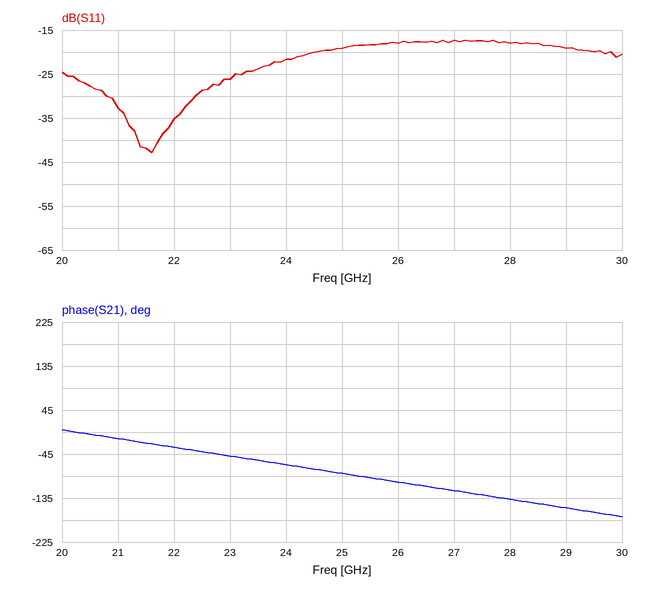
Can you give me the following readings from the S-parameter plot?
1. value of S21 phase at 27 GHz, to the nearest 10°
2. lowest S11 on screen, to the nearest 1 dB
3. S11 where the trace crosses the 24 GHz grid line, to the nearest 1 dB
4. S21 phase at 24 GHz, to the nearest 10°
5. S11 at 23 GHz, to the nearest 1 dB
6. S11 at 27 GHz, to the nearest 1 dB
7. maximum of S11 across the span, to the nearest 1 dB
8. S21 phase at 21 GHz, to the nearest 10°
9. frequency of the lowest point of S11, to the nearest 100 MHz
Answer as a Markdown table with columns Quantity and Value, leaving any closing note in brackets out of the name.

| Quantity | Value |
|---|---|
| value of S21 phase at 27 GHz, to the nearest 10° | -120° |
| lowest S11 on screen, to the nearest 1 dB | -43 dB |
| S11 where the trace crosses the 24 GHz grid line, to the nearest 1 dB | -22 dB |
| S21 phase at 24 GHz, to the nearest 10° | -70° |
| S11 at 23 GHz, to the nearest 1 dB | -26 dB |
| S11 at 27 GHz, to the nearest 1 dB | -17 dB |
| maximum of S11 across the span, to the nearest 1 dB | -17 dB |
| S21 phase at 21 GHz, to the nearest 10° | -10° |
| frequency of the lowest point of S11, to the nearest 100 MHz | 21.6 GHz |
